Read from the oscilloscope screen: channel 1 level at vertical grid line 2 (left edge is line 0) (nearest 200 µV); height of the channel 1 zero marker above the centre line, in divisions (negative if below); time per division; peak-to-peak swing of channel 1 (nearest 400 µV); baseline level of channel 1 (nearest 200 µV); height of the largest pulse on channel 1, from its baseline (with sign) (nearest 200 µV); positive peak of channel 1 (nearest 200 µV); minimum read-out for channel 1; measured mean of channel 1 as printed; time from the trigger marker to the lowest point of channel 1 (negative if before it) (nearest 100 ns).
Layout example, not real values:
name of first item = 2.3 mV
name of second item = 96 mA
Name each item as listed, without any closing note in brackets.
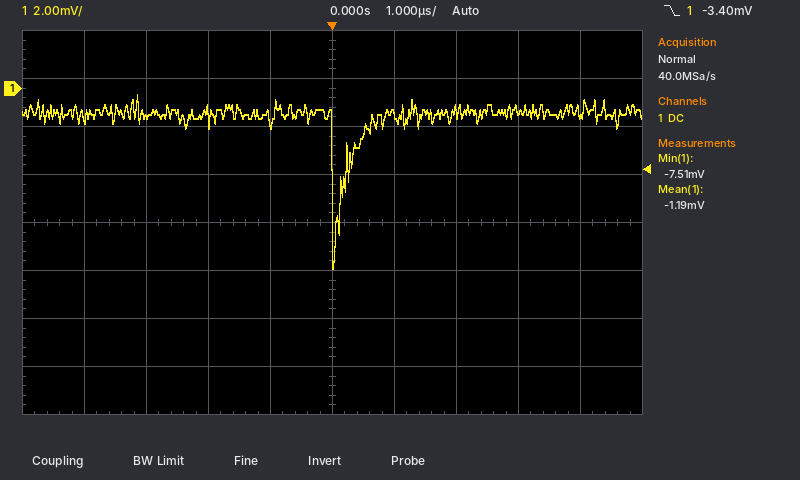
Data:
channel 1 level at vertical grid line 2 (left edge is line 0) = -1.2 mV
height of the channel 1 zero marker above the centre line, in divisions = +2.8 div
time per division = 1 µs
peak-to-peak swing of channel 1 = 7.2 mV
baseline level of channel 1 = -1.0 mV
height of the largest pulse on channel 1, from its baseline (with sign) = -6.4 mV
positive peak of channel 1 = -200 µV
minimum read-out for channel 1 = -7.51 mV
measured mean of channel 1 as printed = -1.19 mV
time from the trigger marker to the lowest point of channel 1 (negative if before it) = 0.0 µs
